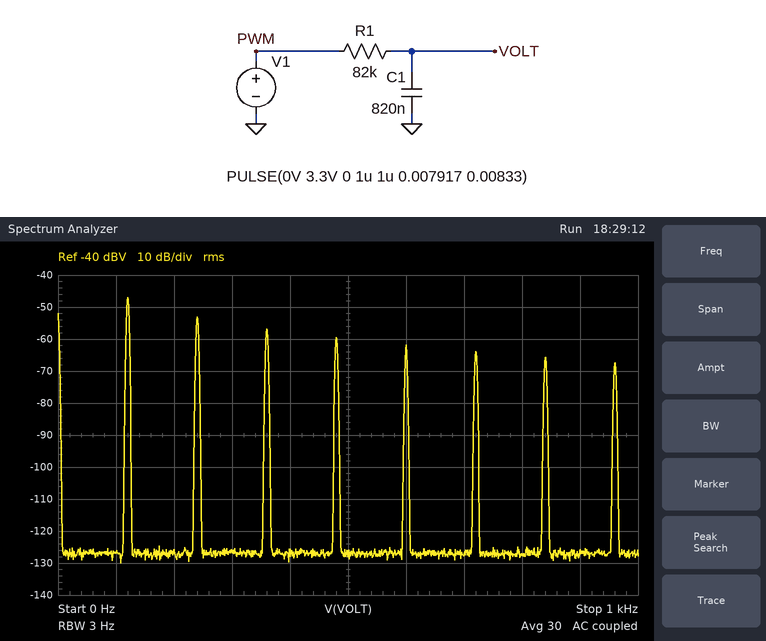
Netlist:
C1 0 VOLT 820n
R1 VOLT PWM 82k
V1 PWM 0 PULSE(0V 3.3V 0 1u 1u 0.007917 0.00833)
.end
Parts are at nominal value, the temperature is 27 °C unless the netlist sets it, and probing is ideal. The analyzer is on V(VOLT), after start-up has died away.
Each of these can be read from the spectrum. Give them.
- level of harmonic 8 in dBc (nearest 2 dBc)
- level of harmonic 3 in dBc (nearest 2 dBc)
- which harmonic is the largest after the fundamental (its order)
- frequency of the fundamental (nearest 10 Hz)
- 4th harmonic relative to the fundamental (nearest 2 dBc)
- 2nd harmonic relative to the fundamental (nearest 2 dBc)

-20 dBc
-10 dBc
2
120 Hz
-12 dBc
-6 dBc
